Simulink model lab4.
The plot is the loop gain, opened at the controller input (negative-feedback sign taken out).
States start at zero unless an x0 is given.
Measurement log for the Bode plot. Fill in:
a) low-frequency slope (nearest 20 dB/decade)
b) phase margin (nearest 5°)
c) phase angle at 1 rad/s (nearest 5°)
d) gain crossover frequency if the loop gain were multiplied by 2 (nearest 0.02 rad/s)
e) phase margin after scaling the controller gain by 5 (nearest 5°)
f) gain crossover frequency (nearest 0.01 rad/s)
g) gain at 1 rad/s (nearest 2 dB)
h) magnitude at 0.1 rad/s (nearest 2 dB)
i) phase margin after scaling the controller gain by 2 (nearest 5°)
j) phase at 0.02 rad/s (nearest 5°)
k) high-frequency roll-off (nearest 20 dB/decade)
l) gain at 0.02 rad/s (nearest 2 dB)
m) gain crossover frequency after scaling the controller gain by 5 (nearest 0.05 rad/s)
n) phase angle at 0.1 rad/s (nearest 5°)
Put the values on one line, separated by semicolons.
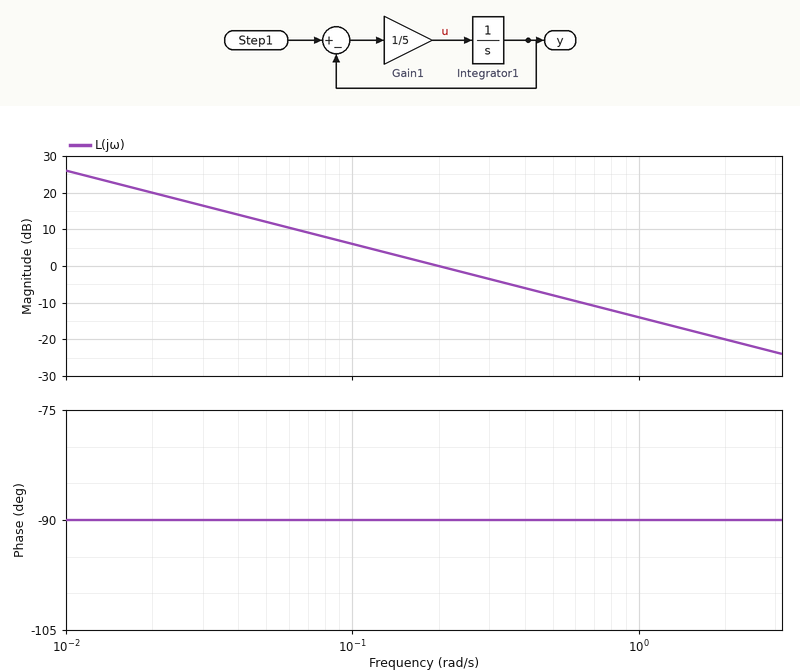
-20 dB/decade; 90°; -90°; 0.40 rad/s; 90°; 0.20 rad/s; -14 dB; 6 dB; 90°; -90°; -20 dB/decade; 20 dB; 1.00 rad/s; -90°
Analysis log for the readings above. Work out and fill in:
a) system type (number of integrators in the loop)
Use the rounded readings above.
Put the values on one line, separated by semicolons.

1
